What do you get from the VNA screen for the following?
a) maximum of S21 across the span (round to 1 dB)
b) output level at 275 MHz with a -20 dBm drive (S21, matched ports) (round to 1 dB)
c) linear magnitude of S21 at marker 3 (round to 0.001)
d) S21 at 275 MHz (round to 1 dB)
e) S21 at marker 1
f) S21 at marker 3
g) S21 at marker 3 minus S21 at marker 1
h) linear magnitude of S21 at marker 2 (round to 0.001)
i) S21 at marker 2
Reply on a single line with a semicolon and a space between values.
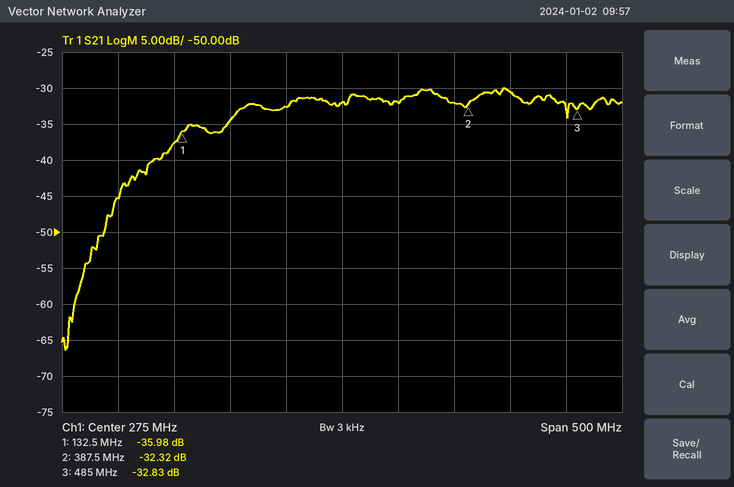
-30 dB; -52 dBm; 0.023; -32 dB; -35.98 dB; -32.83 dB; 3.15 dB; 0.024; -32.32 dB
